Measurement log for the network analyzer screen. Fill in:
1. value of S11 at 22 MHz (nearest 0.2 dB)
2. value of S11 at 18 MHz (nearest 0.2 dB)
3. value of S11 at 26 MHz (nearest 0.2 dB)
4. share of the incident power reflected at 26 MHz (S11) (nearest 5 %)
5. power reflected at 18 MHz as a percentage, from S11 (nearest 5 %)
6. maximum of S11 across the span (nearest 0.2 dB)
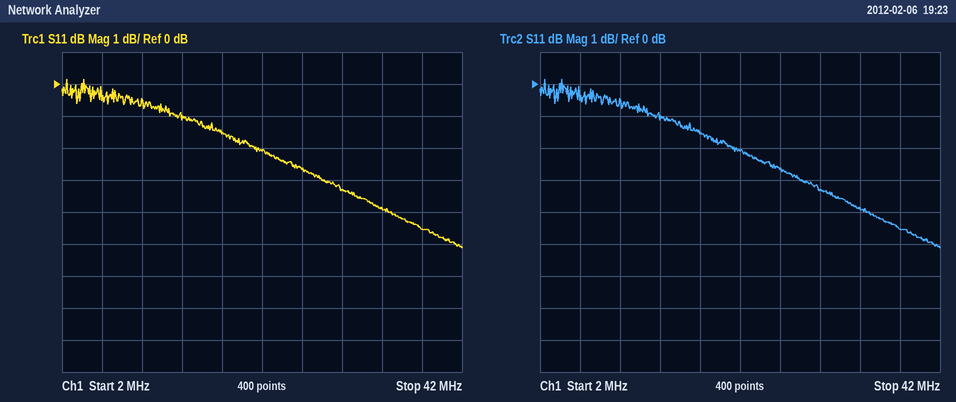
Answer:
-2.0 dB
-1.6 dB
-2.6 dB
55 %
70 %
0.2 dB
